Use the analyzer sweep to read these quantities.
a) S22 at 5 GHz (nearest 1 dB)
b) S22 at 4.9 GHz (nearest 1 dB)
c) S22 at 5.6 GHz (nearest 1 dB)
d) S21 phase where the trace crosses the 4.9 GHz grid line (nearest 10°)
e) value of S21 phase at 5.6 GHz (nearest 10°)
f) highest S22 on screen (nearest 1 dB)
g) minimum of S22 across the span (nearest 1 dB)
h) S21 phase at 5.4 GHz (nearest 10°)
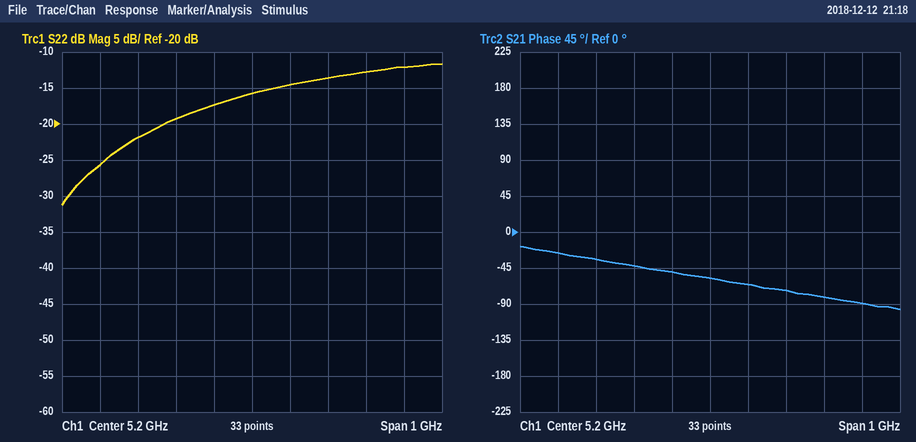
-19 dB
-22 dB
-12 dB
-30°
-90°
-12 dB
-31 dB
-70°
